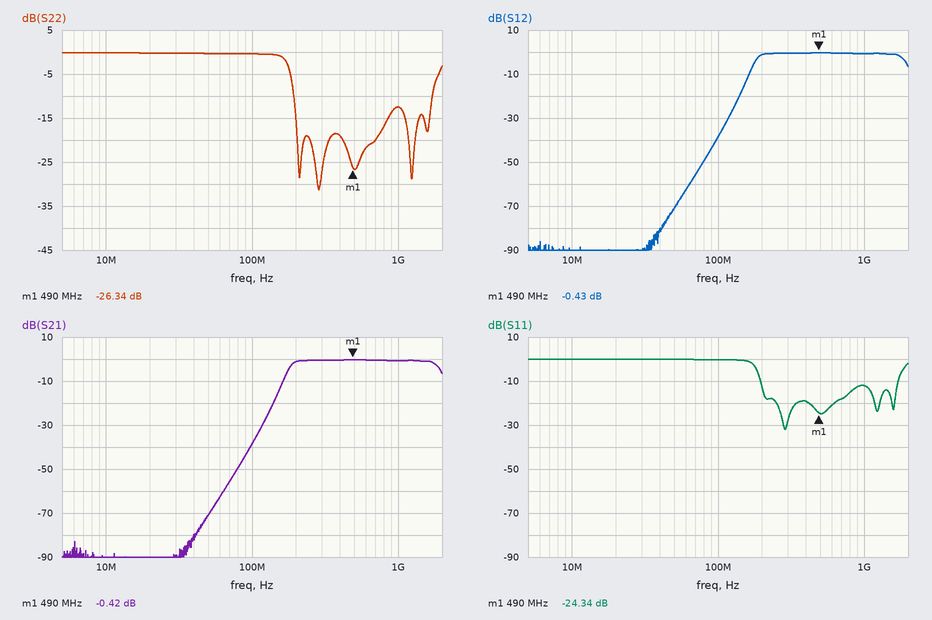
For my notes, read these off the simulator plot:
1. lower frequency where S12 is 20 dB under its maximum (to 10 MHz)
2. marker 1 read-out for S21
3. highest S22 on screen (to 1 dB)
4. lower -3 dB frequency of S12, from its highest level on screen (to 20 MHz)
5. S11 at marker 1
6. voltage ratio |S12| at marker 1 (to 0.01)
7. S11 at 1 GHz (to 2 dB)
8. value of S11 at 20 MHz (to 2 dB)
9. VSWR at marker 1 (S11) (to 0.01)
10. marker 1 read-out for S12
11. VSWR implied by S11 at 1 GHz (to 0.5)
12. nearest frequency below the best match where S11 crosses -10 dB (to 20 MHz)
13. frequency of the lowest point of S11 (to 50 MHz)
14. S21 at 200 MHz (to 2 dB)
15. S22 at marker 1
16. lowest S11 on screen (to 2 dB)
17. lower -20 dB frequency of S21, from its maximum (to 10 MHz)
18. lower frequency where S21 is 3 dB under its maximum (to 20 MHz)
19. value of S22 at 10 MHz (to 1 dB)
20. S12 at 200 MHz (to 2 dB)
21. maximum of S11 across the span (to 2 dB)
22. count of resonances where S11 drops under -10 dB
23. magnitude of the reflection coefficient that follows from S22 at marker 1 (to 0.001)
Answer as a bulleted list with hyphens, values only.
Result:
- 140 MHz
- -0.42 dB
- 0 dB
- 180 MHz
- -24.34 dB
- 0.95
- -12 dB
- 0 dB
- 1.13
- -0.43 dB
- 1.5
- 200 MHz
- 300 MHz
- -2 dB
- -26.34 dB
- -32 dB
- 140 MHz
- 180 MHz
- 0 dB
- -2 dB
- 0 dB
- 4
- 0.048
